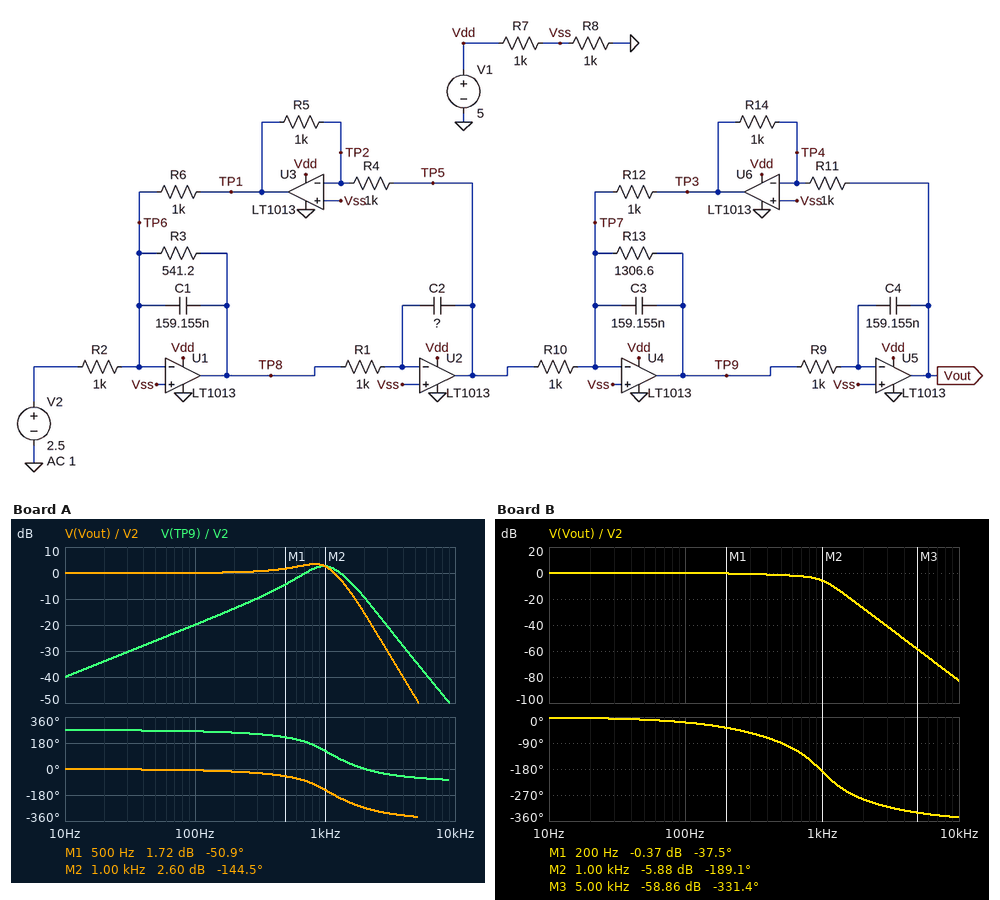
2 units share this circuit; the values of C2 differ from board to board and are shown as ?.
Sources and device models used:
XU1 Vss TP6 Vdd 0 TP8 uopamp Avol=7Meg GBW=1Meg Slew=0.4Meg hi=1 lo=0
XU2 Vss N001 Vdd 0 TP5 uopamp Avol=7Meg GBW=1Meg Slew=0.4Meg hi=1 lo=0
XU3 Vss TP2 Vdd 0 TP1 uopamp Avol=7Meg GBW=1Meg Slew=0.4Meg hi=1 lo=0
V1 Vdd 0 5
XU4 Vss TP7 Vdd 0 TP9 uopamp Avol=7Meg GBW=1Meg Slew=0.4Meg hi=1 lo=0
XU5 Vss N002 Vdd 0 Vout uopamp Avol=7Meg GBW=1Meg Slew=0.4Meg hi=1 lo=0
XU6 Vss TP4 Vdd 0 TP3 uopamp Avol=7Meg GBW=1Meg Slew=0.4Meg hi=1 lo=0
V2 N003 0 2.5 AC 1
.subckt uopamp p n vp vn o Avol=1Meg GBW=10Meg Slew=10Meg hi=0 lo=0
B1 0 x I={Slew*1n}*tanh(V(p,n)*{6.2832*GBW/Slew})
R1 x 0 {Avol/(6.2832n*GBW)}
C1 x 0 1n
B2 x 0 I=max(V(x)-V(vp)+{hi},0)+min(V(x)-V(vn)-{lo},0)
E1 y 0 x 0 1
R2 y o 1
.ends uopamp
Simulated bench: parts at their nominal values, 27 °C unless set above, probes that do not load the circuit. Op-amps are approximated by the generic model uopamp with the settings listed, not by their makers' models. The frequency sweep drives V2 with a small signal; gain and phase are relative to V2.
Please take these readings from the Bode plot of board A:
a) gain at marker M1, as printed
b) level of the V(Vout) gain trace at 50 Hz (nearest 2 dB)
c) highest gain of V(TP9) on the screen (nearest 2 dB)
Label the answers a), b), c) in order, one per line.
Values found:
a) 1.72 dB
b) 0 dB
c) 2 dB
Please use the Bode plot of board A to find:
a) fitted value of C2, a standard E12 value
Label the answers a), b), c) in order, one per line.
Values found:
a) 68 nF
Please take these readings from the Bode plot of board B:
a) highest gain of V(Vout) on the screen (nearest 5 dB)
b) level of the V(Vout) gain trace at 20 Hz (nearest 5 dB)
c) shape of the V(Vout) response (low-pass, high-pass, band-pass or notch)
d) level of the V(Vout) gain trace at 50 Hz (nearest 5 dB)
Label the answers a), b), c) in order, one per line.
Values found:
a) 0 dB
b) 0 dB
c) low-pass
d) 0 dB
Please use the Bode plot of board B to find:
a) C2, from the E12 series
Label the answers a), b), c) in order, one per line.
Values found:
a) 220 nF
